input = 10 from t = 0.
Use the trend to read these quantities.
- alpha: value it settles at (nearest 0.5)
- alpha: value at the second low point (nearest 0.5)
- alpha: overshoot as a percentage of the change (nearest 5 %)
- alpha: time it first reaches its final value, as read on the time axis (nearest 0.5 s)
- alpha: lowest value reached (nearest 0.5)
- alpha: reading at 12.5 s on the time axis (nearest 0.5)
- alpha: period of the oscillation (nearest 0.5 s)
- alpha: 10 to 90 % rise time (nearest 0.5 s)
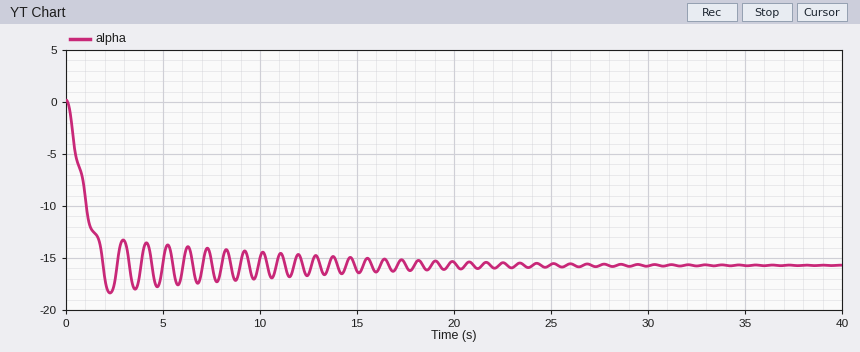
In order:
-15.5
-18.0
15 %
2.0 s
-18.5
-16.5
1.5 s
1.5 s
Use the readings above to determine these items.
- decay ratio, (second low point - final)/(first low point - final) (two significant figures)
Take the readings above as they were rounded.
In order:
0.83
